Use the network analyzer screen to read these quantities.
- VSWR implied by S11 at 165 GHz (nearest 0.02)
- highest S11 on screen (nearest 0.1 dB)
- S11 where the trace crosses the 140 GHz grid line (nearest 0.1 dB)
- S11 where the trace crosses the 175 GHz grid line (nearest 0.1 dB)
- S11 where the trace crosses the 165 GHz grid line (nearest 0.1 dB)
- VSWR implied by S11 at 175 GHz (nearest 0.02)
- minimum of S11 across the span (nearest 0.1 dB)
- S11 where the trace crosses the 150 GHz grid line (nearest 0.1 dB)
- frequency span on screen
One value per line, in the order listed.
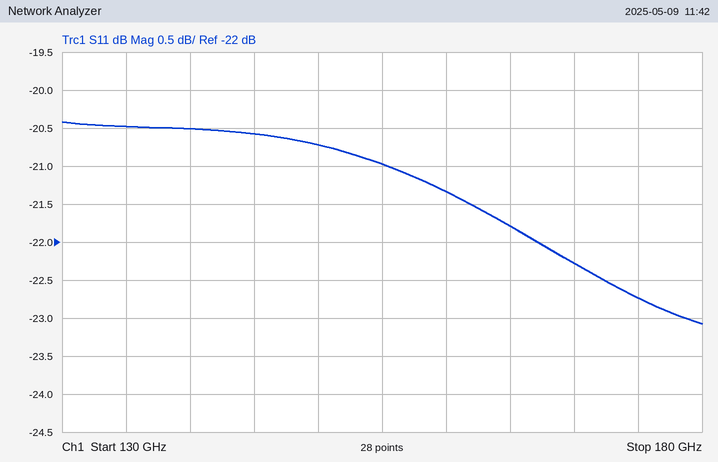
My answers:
1.18
-20.4 dB
-20.5 dB
-22.7 dB
-21.8 dB
1.16
-23.1 dB
-20.7 dB
50 GHz
